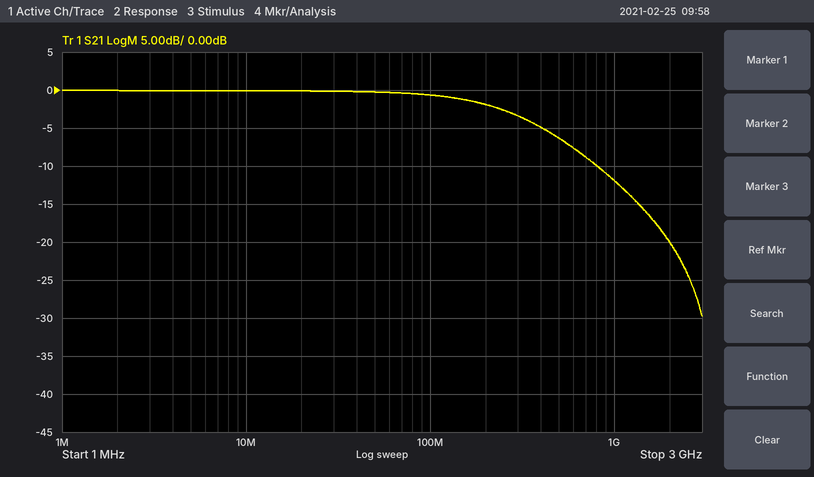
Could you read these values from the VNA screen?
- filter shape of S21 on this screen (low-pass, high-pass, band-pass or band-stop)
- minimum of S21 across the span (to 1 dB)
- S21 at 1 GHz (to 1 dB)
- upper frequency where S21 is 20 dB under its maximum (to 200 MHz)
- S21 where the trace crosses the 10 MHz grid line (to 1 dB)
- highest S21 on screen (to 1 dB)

low-pass
-30 dB
-12 dB
2.0 GHz
0 dB
0 dB
